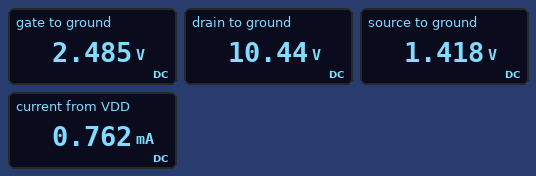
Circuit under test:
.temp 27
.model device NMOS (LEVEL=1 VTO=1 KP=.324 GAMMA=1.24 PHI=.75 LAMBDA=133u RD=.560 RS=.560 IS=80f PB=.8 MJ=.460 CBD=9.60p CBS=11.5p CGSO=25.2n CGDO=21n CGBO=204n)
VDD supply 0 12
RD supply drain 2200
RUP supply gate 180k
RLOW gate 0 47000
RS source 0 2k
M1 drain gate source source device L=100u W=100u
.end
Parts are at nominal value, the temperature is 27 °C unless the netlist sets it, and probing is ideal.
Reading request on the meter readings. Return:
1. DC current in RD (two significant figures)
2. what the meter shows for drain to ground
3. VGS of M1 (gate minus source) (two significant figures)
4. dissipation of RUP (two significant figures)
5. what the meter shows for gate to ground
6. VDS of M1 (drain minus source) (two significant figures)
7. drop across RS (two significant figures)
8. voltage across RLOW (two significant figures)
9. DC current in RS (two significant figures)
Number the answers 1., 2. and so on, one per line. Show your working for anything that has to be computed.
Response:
1. (12 V - 10.44 V) / 2.2 kΩ = 710 µA
2. 10.44 V
3. 2.485 V - 1.418 V = 1.1 V
4. (12 V - 2.485 V)^2 / 180 kΩ = 500 µW
5. 2.485 V
6. 10.44 V - 1.418 V = 9.0 V
7. 1.418 V = 1.4 V
8. 2.485 V = 2.5 V
9. (1.418 V) / 2 kΩ = 710 µA
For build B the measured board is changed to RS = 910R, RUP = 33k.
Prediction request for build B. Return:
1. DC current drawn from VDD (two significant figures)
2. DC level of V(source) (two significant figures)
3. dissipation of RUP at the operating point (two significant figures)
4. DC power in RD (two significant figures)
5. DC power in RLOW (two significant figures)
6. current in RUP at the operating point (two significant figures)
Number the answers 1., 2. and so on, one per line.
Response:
1. 4.0 mA
2. 3.5 V
3. 740 µW
4. 33 mW
5. 1.1 mW
6. 150 µA
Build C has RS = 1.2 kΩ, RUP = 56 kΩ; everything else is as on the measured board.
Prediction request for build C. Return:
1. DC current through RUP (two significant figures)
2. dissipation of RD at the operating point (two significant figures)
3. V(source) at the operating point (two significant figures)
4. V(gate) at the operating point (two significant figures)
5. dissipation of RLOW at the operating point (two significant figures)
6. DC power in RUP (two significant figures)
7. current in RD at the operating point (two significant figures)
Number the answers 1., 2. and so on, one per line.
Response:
1. 120 µA
2. 27 mW
3. 4.2 V
4. 5.5 V
5. 640 µW
6. 760 µW
7. 3.5 mA
